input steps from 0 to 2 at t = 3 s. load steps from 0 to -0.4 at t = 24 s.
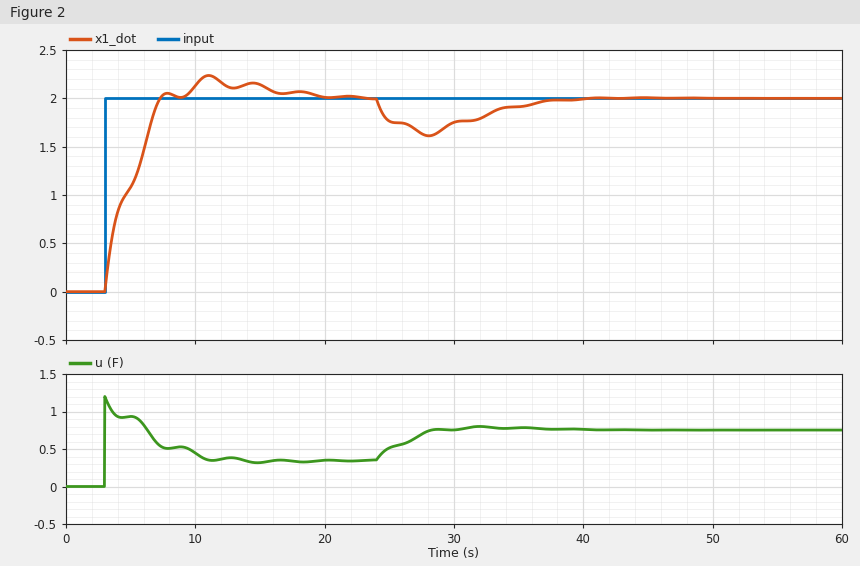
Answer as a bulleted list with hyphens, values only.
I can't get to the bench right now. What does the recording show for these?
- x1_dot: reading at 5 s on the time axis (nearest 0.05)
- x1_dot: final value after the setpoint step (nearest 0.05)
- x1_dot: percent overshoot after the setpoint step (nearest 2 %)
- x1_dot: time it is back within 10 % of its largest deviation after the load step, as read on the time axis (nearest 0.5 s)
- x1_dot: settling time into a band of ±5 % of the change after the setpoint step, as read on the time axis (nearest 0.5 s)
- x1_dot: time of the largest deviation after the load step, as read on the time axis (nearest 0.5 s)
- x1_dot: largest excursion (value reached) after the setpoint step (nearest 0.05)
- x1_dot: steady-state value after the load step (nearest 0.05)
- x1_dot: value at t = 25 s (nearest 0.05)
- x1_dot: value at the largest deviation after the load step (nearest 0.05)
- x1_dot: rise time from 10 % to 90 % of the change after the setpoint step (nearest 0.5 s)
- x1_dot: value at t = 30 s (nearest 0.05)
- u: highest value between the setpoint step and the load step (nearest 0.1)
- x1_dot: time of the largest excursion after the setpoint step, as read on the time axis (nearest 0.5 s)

- 1.10
- 2.00
- 12 %
- 36.5 s
- 15.5 s
- 28.0 s
- 2.25
- 2.00
- 1.75
- 1.60
- 3.5 s
- 1.75
- 1.2
- 11.0 s
